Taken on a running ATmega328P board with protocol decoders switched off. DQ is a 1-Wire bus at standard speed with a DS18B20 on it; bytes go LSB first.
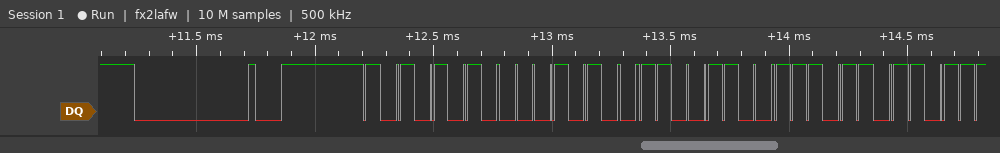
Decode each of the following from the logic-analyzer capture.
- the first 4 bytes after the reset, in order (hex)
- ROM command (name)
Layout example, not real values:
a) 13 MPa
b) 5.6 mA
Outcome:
a) 55 28 33 B7
b) Match ROM
